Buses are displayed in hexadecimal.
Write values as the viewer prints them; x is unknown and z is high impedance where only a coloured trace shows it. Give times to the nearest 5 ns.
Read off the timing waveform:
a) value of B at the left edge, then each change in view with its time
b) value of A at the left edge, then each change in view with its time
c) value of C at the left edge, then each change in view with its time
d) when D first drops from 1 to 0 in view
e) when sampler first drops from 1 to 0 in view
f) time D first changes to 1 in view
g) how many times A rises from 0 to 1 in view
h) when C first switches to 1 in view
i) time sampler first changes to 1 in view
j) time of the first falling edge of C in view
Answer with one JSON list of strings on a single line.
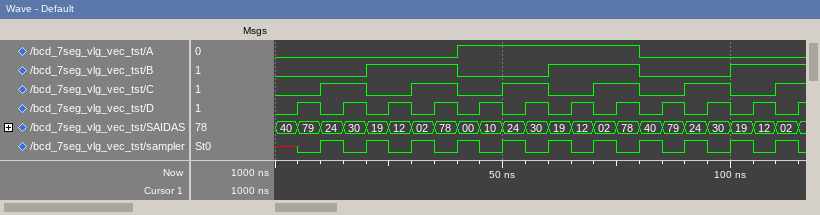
["0, 1 at 20 ns, 0 at 40 ns, 1 at 60 ns, 0 at 80 ns, 1 at 100 ns", "0, 1 at 40 ns, 0 at 80 ns", "0, 1 at 10 ns, 0 at 20 ns, 1 at 30 ns, 0 at 40 ns, 1 at 50 ns, 0 at 60 ns, 1 at 70 ns, 0 at 80 ns, 1 at 90 ns, 0 at 100 ns, 1 at 110 ns", "10 ns", "15 ns", "5 ns", "1", "10 ns", "10 ns", "20 ns"]
